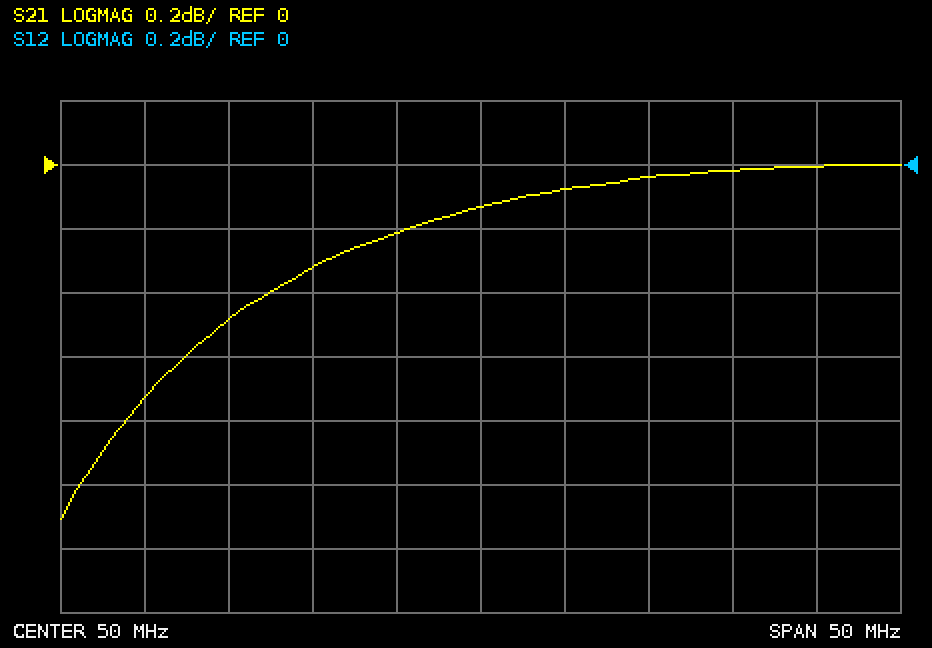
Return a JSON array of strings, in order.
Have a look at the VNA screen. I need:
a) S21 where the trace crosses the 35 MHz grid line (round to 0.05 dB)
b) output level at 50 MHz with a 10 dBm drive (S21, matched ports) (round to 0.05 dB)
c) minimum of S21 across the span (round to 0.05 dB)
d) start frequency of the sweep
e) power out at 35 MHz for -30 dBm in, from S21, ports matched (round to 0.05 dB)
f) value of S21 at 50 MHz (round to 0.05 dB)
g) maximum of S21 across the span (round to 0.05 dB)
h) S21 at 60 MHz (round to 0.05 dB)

["-0.50 dB", "9.85 dBm", "-1.10 dB", "25 MHz", "-30.50 dBm", "-0.15 dB", "0.00 dB", "-0.05 dB"]
